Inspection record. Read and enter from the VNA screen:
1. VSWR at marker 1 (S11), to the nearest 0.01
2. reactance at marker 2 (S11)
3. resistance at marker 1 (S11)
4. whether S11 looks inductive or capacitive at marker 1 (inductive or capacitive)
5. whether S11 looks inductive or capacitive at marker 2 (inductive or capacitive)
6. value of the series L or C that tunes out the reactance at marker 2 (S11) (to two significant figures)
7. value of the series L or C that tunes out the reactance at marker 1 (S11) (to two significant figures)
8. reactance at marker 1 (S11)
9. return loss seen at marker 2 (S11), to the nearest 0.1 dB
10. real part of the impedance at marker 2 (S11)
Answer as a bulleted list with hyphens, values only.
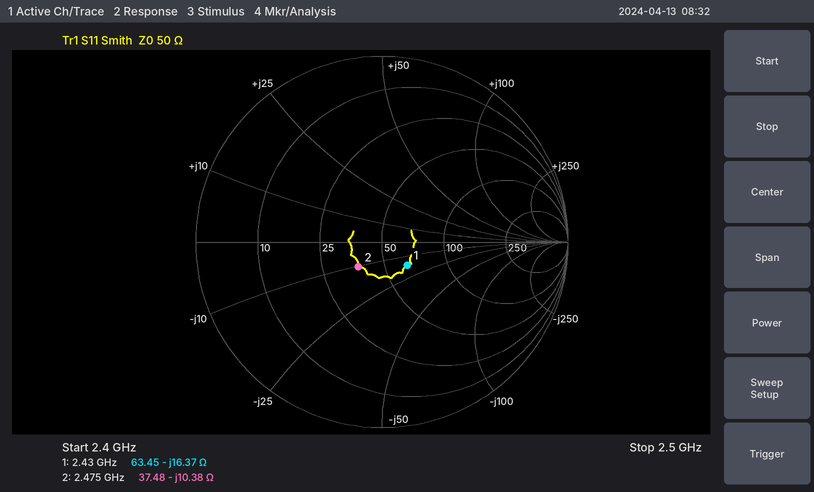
- 1.45
- -10.38 Ω
- 63.45 Ω
- capacitive
- capacitive
- 670 pH
- 1.1 nH
- -16.37 Ω
- 14.7 dB
- 37.48 Ω
